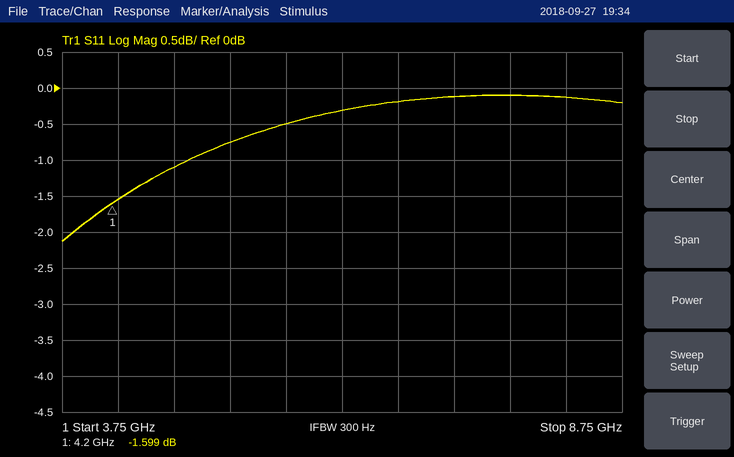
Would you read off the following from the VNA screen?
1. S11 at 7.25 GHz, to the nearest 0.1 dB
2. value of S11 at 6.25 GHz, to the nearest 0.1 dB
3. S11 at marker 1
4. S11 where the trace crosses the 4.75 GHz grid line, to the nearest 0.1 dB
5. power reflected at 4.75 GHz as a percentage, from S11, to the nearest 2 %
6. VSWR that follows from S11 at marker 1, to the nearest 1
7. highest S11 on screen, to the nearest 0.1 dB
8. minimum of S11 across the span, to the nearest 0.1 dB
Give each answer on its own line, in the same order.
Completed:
-0.1 dB
-0.3 dB
-1.599 dB
-1.1 dB
78 %
11
-0.1 dB
-2.1 dB
